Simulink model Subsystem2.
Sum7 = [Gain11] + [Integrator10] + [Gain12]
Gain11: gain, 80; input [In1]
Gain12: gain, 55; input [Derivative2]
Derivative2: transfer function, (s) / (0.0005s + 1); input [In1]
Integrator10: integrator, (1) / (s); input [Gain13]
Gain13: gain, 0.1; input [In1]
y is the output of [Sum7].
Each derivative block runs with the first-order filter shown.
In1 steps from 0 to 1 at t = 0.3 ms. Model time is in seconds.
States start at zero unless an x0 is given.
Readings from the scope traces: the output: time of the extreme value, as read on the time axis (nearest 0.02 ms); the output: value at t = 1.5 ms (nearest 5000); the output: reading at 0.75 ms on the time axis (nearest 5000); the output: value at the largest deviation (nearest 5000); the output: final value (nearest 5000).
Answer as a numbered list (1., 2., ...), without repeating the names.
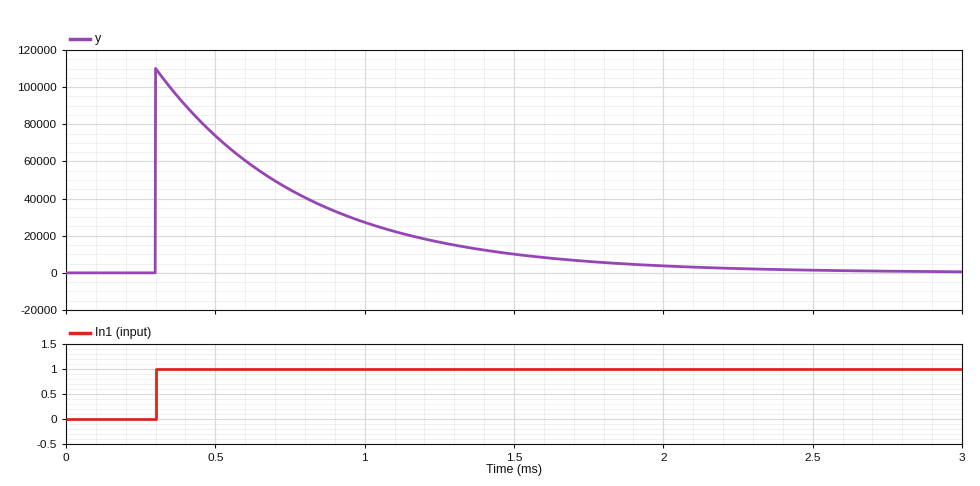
1. 0.30 ms
2. 10000
3. 45000
4. 110000
5. 0
